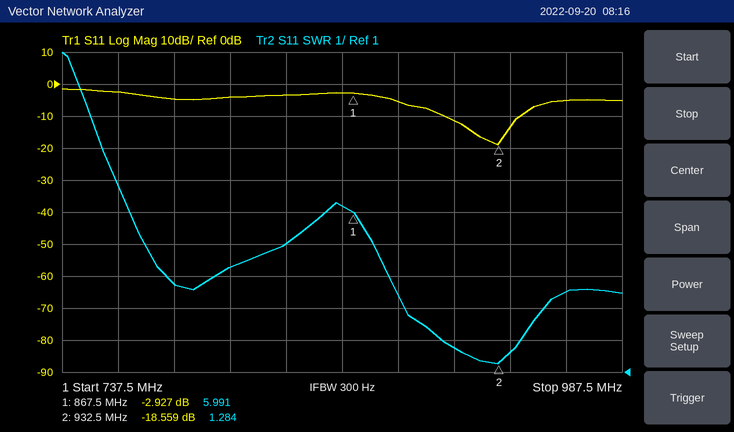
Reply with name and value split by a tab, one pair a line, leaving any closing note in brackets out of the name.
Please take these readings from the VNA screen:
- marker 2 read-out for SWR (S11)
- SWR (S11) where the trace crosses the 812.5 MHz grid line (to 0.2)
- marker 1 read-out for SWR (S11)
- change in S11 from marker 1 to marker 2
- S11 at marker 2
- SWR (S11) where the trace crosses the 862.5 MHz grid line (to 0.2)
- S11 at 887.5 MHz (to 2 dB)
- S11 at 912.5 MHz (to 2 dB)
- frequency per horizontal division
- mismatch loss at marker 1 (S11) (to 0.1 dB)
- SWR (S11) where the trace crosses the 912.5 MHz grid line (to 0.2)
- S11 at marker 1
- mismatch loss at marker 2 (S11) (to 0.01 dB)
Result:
marker 2 read-out for SWR	1.284
SWR (S11) where the trace crosses the 812.5 MHz grid line	4.2
marker 1 read-out for SWR	5.991
change in S11 from marker 1 to marker 2	-15.632 dB
S11 at marker 2	-18.559 dB
SWR (S11) where the trace crosses the 862.5 MHz grid line	6.2
S11 at 887.5 MHz	-6 dB
S11 at 912.5 MHz	-12 dB
frequency per horizontal division	25 MHz
mismatch loss at marker 1 (S11)	3.1 dB
SWR (S11) where the trace crosses the 912.5 MHz grid line	1.8
S11 at marker 1	-2.927 dB
mismatch loss at marker 2 (S11)	0.06 dB
